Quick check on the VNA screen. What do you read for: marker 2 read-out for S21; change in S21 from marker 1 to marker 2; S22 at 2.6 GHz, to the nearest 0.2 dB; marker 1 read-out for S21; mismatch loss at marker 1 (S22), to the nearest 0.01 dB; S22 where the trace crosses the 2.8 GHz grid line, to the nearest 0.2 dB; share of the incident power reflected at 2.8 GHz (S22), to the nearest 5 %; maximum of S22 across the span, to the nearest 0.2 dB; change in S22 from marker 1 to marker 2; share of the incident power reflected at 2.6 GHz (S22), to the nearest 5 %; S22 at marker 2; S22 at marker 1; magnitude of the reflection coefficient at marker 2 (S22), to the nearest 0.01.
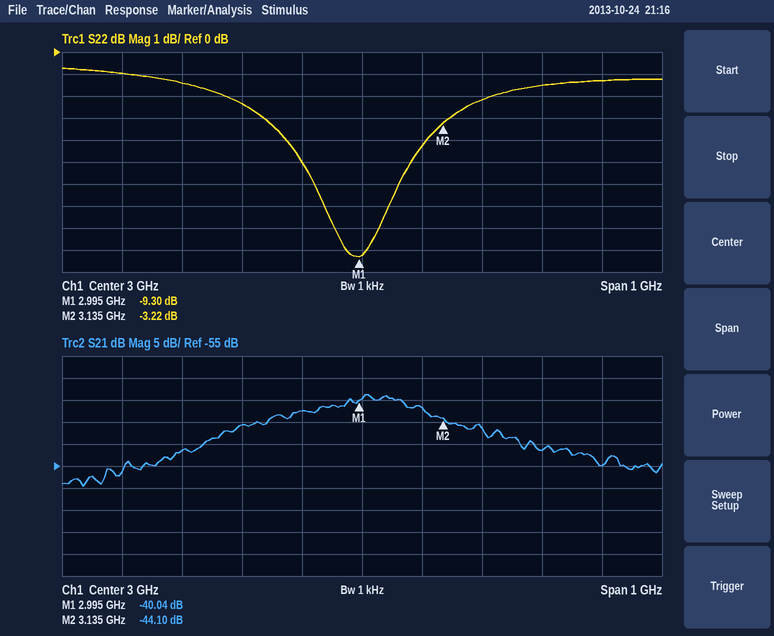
-44.10 dB
-4.06 dB
-1.0 dB
-40.04 dB
0.54 dB
-2.4 dB
60 %
-0.8 dB
6.08 dB
80 %
-3.22 dB
-9.30 dB
0.69
